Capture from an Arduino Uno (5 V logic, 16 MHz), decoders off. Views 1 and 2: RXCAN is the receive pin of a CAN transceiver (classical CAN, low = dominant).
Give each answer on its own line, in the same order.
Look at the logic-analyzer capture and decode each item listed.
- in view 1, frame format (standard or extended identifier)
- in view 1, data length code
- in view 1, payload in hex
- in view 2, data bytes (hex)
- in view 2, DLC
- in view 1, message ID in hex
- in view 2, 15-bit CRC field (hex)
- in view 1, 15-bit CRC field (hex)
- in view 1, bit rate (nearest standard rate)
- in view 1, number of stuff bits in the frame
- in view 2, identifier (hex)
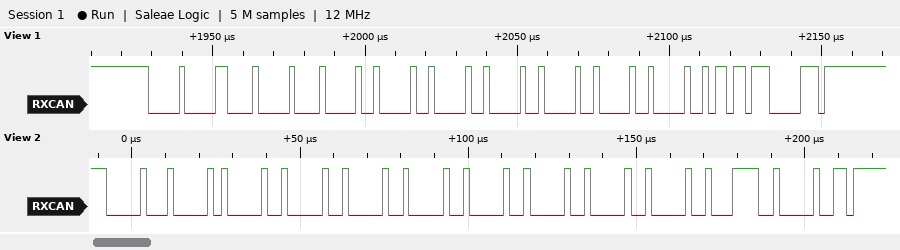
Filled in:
standard
8
02 02 02 02 02 02 02 02
08 08 08 08 08 08 08 08
8
0x002
0x7901
0x6DC1
500 kbit/s
11
0x008
